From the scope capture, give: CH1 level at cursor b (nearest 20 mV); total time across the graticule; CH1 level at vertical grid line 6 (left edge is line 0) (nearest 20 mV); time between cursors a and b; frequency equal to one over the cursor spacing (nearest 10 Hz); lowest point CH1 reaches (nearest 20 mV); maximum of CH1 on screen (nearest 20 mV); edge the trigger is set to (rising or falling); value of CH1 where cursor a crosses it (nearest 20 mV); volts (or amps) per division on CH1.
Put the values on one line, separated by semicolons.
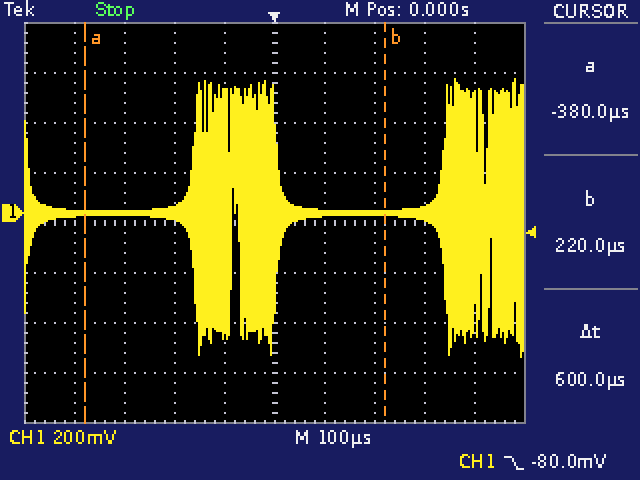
0 mV; 1 ms; 0 mV; 600 µs; 1.67 kHz; -580 mV; 540 mV; falling; 0 mV; 200 mV
